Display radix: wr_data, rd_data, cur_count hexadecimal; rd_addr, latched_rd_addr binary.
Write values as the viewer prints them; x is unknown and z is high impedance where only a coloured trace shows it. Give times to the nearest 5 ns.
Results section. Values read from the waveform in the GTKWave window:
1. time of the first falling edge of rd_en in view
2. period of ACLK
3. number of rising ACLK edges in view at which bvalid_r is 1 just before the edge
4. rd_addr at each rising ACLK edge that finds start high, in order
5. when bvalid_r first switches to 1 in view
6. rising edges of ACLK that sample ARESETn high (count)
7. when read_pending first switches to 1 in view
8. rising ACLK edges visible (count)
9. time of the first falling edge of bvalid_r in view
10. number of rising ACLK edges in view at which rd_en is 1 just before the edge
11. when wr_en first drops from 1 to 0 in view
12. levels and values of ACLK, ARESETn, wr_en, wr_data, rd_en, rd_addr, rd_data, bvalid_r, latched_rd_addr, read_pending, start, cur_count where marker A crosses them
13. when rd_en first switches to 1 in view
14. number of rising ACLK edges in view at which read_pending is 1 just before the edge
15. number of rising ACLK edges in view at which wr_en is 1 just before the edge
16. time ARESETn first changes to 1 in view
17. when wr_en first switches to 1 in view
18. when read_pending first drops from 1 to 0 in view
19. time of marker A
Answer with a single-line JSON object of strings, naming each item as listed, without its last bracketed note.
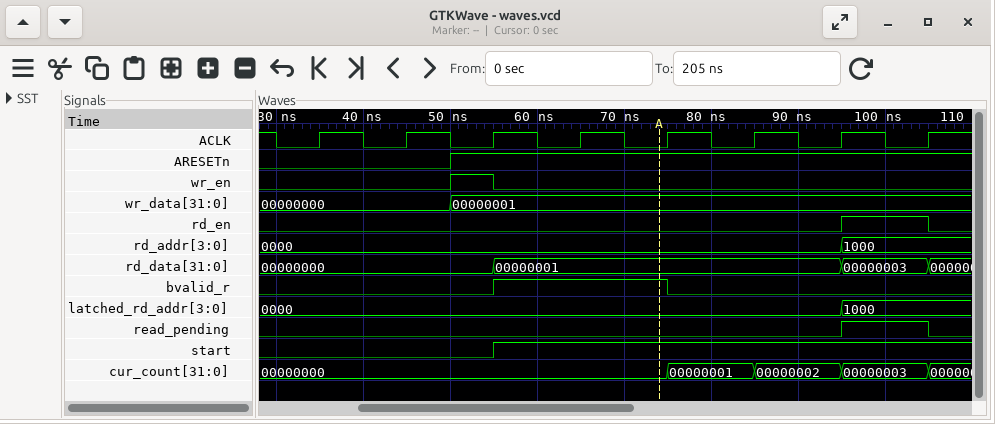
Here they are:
{"time of the first falling edge of rd_en in view": "105 ns", "period of ACLK": "10 ns", "number of rising ACLK edges in view at which bvalid_r is 1 just before the edge": "2", "rd_addr at each rising ACLK edge that finds start high, in order": "0000, 0000, 0000, 0000, 1000", "when bvalid_r first switches to 1 in view": "55 ns", "rising edges of ACLK that sample ARESETn high": "6", "when read_pending first switches to 1 in view": "95 ns", "rising ACLK edges visible": "8", "time of the first falling edge of bvalid_r in view": "75 ns", "number of rising ACLK edges in view at which rd_en is 1 just before the edge": "1", "when wr_en first drops from 1 to 0 in view": "55 ns", "levels and values of ACLK, ARESETn, wr_en, wr_data, rd_en, rd_addr, rd_data, bvalid_r, latched_rd_addr, read_pending, start, cur_count where marker A crosses them": "ACLK=0, ARESETn=1, wr_en=0, wr_data=00000001, rd_en=0, rd_addr=0000, rd_data=00000001, bvalid_r=1, latched_rd_addr=0000, read_pending=0, start=1, cur_count=00000000", "when rd_en first switches to 1 in view": "95 ns", "number of rising ACLK edges in view at which read_pending is 1 just before the edge": "1", "number of rising ACLK edges in view at which wr_en is 1 just before the edge": "1", "time ARESETn first changes to 1 in view": "50 ns", "when wr_en first switches to 1 in view": "50 ns", "when read_pending first drops from 1 to 0 in view": "105 ns", "time of marker A": "75 ns"}
